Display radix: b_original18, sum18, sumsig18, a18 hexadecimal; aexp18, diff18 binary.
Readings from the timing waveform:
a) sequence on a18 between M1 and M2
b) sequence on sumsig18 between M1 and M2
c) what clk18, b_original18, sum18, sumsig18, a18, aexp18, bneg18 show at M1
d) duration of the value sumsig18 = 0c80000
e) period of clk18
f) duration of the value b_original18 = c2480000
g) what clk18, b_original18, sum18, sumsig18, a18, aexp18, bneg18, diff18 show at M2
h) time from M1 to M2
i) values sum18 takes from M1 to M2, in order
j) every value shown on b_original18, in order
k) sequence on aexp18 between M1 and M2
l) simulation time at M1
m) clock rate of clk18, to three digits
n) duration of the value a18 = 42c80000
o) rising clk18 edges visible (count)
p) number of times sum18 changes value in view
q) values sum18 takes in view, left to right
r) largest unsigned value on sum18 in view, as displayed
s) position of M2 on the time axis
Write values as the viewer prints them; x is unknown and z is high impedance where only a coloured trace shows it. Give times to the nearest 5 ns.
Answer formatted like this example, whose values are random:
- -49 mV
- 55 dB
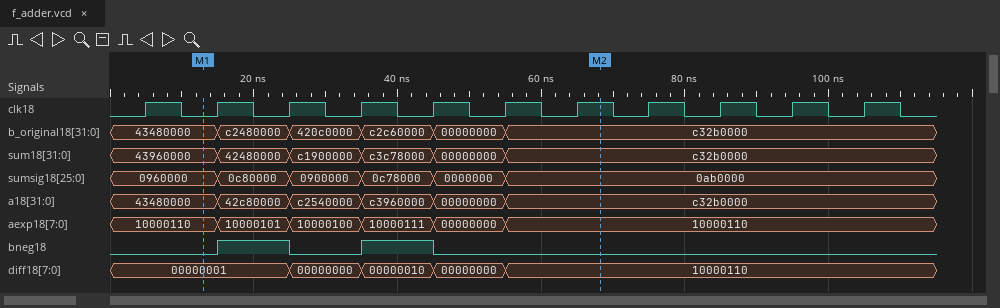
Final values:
- 43480000, 42c80000, c2540000, c3960000, 00000000, c32b0000
- 0960000, 0c80000, 0900000, 0c78000, 0000000, 0ab0000
- clk18=0, b_original18=43480000, sum18=43960000, sumsig18=0960000, a18=43480000, aexp18=10000110, bneg18=0
- 10 ns
- 10 ns
- 10 ns
- clk18=1, b_original18=c32b0000, sum18=c32b0000, sumsig18=0ab0000, a18=c32b0000, aexp18=10000110, bneg18=0, diff18=10000110
- 55 ns
- 43960000, 42480000, c1900000, c3c78000, 00000000, c32b0000
- 43480000, c2480000, 420c0000, c2c60000, 00000000, c32b0000
- 10000110, 10000101, 10000100, 10000111, 00000000, 10000110
- 15 ns
- 100 MHz
- 10 ns
- 11
- 5
- 43960000, 42480000, c1900000, c3c78000, 00000000, c32b0000
- c3c78000
- 70 ns
